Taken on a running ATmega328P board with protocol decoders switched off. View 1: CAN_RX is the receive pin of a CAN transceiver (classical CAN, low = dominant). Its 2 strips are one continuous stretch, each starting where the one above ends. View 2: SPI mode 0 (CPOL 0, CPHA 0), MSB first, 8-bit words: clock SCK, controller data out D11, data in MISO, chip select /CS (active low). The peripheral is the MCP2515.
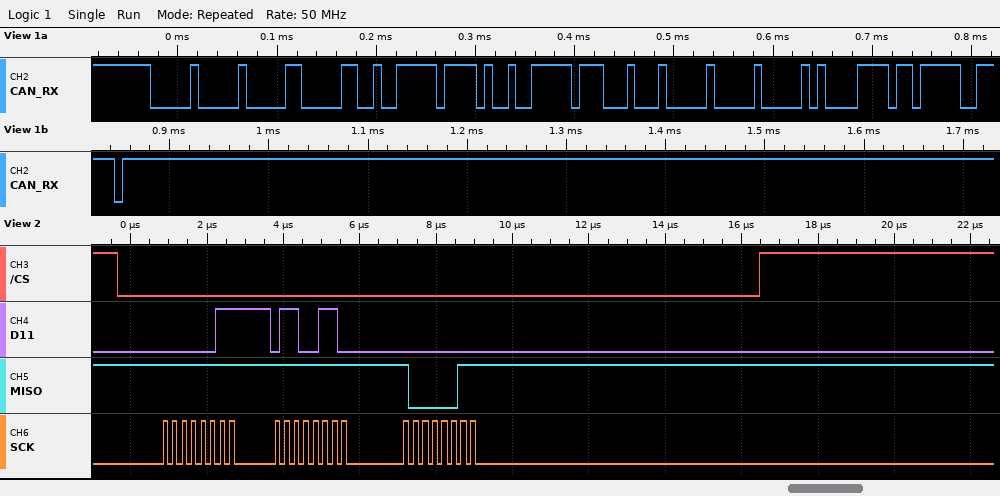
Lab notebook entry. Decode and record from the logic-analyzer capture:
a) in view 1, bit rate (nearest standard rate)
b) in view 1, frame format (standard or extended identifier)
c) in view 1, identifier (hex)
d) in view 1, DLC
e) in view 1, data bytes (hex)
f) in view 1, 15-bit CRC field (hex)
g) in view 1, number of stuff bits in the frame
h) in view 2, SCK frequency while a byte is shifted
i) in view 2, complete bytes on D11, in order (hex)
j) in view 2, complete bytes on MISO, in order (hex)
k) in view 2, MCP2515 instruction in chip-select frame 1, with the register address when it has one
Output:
125 kbit/s
standard
0x000
8
24 FF A4 FF 11 00 00 87
0x5BEF
10
4 MHz
03 66 00
FF FF 83
READ 0x66
